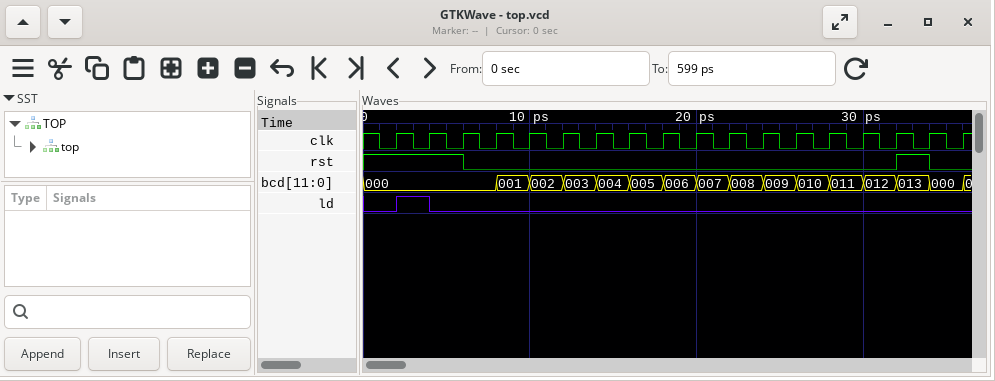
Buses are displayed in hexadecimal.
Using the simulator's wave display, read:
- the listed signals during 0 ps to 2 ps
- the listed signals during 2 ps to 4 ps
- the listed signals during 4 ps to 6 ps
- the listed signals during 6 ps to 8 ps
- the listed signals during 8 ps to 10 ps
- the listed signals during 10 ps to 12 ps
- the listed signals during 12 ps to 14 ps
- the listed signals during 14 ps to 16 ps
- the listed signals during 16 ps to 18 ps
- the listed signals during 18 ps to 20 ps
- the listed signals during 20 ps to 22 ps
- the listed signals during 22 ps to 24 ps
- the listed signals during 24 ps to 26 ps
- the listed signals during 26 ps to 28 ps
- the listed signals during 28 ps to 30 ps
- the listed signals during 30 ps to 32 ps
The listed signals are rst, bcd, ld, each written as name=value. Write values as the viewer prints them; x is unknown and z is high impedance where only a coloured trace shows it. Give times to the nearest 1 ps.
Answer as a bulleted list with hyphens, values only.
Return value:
- rst=1, bcd=000, ld=0
- rst=1, bcd=000, ld=1
- rst=1, bcd=000, ld=0
- rst=0, bcd=000, ld=0
- rst=0, bcd=001, ld=0
- rst=0, bcd=002, ld=0
- rst=0, bcd=003, ld=0
- rst=0, bcd=004, ld=0
- rst=0, bcd=005, ld=0
- rst=0, bcd=006, ld=0
- rst=0, bcd=007, ld=0
- rst=0, bcd=008, ld=0
- rst=0, bcd=009, ld=0
- rst=0, bcd=010, ld=0
- rst=0, bcd=011, ld=0
- rst=0, bcd=012, ld=0
